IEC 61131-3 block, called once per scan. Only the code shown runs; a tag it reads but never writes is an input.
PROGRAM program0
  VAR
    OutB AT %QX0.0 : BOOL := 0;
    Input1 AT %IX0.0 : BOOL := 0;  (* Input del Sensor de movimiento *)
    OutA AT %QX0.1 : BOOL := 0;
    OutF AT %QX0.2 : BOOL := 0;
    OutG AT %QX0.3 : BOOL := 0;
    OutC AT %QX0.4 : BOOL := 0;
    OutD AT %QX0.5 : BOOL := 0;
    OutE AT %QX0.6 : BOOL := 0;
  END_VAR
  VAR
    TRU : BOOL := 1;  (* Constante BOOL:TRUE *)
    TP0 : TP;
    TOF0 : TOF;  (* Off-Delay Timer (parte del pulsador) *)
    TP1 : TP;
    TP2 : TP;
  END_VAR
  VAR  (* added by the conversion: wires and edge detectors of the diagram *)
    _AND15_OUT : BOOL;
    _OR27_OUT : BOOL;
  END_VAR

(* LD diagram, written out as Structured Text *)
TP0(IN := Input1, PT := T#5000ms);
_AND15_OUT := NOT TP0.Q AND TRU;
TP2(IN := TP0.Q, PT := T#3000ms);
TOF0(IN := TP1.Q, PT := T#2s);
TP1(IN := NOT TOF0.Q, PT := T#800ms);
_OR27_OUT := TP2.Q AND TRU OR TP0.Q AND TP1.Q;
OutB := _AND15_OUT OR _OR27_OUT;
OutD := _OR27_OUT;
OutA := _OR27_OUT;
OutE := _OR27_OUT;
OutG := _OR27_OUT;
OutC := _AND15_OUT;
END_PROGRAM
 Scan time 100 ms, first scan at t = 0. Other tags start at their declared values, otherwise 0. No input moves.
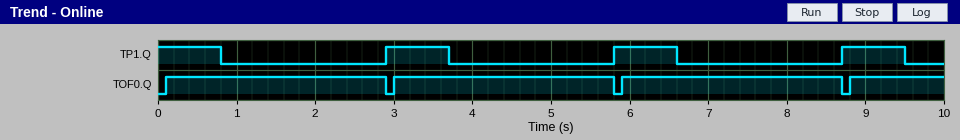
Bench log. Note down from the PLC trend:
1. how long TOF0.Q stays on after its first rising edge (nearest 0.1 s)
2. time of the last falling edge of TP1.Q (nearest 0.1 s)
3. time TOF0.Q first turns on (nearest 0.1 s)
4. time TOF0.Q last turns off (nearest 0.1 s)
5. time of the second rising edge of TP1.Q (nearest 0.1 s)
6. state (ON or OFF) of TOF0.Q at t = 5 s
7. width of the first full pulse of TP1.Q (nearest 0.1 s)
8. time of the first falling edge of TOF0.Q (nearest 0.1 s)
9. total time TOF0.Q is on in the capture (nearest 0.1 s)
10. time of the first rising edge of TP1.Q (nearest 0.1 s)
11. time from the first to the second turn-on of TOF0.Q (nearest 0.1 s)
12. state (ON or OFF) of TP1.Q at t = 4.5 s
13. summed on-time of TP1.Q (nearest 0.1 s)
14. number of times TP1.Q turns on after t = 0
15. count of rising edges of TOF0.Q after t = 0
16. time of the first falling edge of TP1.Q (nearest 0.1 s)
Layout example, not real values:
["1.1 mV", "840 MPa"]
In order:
["2.8 s", "9.5 s", "0.1 s", "8.7 s", "5.8 s", "ON", "0.8 s", "2.9 s", "9.6 s", "2.9 s", "2.9 s", "OFF", "3.2 s", "3", "4", "0.8 s"]
